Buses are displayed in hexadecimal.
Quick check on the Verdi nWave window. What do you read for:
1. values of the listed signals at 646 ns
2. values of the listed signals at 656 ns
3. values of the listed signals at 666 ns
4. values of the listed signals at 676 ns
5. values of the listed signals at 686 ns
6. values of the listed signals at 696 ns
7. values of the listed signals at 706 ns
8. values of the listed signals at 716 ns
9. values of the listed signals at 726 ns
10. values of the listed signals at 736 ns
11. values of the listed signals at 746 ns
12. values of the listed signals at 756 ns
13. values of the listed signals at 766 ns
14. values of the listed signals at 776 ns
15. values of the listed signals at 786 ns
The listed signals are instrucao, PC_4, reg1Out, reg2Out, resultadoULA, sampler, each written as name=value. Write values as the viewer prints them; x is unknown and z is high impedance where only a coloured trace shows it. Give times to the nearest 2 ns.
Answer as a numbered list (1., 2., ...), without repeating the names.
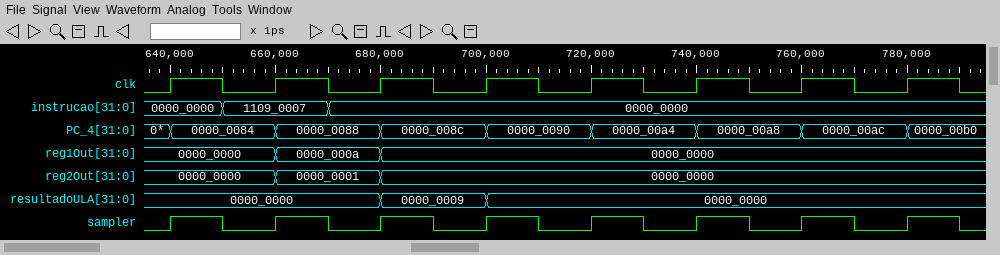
1. instrucao=0000_0000, PC_4=0000_0084, reg1Out=0000_0000, reg2Out=0000_0000, resultadoULA=0000_0000, sampler=1
2. instrucao=1109_0007, PC_4=0000_0084, reg1Out=0000_0000, reg2Out=0000_0000, resultadoULA=0000_0000, sampler=0
3. instrucao=1109_0007, PC_4=0000_0088, reg1Out=0000_000a, reg2Out=0000_0001, resultadoULA=0000_0000, sampler=1
4. instrucao=0000_0000, PC_4=0000_0088, reg1Out=0000_000a, reg2Out=0000_0001, resultadoULA=0000_0000, sampler=0
5. instrucao=0000_0000, PC_4=0000_008c, reg1Out=0000_0000, reg2Out=0000_0000, resultadoULA=0000_0009, sampler=1
6. instrucao=0000_0000, PC_4=0000_008c, reg1Out=0000_0000, reg2Out=0000_0000, resultadoULA=0000_0009, sampler=0
7. instrucao=0000_0000, PC_4=0000_0090, reg1Out=0000_0000, reg2Out=0000_0000, resultadoULA=0000_0000, sampler=1
8. instrucao=0000_0000, PC_4=0000_0090, reg1Out=0000_0000, reg2Out=0000_0000, resultadoULA=0000_0000, sampler=0
9. instrucao=0000_0000, PC_4=0000_00a4, reg1Out=0000_0000, reg2Out=0000_0000, resultadoULA=0000_0000, sampler=1
10. instrucao=0000_0000, PC_4=0000_00a4, reg1Out=0000_0000, reg2Out=0000_0000, resultadoULA=0000_0000, sampler=0
11. instrucao=0000_0000, PC_4=0000_00a8, reg1Out=0000_0000, reg2Out=0000_0000, resultadoULA=0000_0000, sampler=1
12. instrucao=0000_0000, PC_4=0000_00a8, reg1Out=0000_0000, reg2Out=0000_0000, resultadoULA=0000_0000, sampler=0
13. instrucao=0000_0000, PC_4=0000_00ac, reg1Out=0000_0000, reg2Out=0000_0000, resultadoULA=0000_0000, sampler=1
14. instrucao=0000_0000, PC_4=0000_00ac, reg1Out=0000_0000, reg2Out=0000_0000, resultadoULA=0000_0000, sampler=0
15. instrucao=0000_0000, PC_4=0000_00b0, reg1Out=0000_0000, reg2Out=0000_0000, resultadoULA=0000_0000, sampler=1
